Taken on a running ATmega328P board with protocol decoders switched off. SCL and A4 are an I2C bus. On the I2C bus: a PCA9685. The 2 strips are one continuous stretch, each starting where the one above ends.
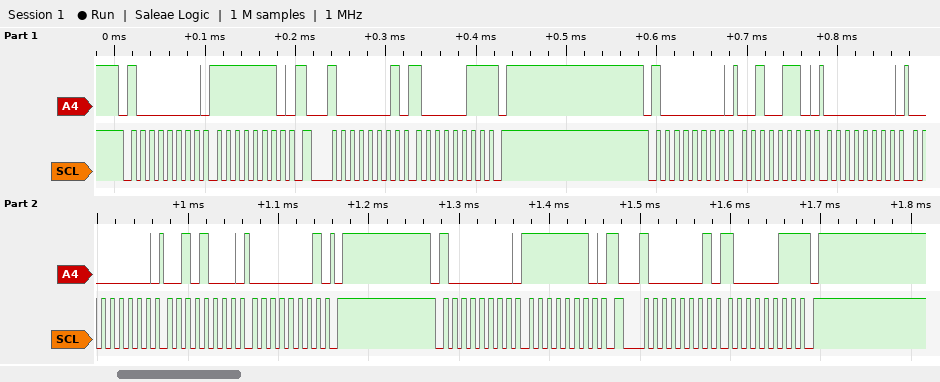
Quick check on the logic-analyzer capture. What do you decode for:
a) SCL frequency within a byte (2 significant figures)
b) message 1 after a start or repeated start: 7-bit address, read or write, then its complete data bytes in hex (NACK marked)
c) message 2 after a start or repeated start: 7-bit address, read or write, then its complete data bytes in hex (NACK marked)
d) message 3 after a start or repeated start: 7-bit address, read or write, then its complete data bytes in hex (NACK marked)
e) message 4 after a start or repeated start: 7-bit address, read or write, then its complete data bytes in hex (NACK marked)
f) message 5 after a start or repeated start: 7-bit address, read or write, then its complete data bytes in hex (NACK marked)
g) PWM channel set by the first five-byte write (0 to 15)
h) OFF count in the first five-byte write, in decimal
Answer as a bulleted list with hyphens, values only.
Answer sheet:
- 100 kHz
- 0x40 write: FE
- 0x40 read: 83 NACK
- 0x40 write: 26 00 00 28 01
- 0x40 write: FE
- 0x40 read: 83 NACK
- 8
- 296
